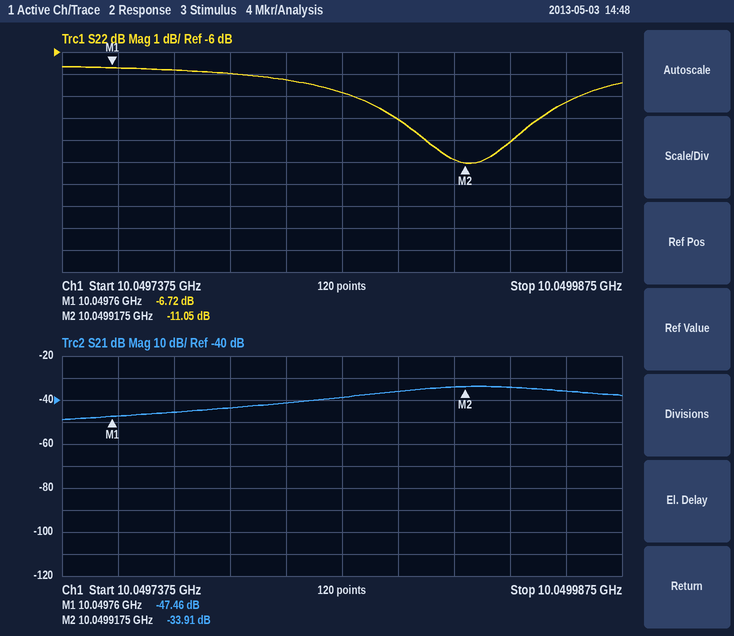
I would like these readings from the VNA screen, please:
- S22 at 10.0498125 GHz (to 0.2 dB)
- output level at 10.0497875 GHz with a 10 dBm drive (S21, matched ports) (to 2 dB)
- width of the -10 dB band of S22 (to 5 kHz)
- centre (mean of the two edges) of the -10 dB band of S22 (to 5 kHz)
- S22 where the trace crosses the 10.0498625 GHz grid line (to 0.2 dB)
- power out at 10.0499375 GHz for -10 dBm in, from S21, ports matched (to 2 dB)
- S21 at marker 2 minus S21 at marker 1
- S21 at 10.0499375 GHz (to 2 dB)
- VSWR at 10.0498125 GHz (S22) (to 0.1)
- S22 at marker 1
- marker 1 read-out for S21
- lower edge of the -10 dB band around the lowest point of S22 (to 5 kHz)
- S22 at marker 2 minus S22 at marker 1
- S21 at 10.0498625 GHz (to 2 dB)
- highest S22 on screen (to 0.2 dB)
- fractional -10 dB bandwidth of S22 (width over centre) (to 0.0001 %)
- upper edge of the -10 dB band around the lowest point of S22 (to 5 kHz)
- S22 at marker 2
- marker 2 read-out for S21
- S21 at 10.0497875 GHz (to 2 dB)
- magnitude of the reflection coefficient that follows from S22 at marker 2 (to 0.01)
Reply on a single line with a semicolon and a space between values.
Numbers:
-7.0 dB; -36 dBm; 40 kHz; 10.049920 GHz; -7.8 dB; -44 dBm; 13.55 dB; -34 dB; 2.6; -6.72 dB; -47.46 dB; 10.049900 GHz; -4.33 dB; -38 dB; -6.6 dB; 0.0004 %; 10.049940 GHz; -11.05 dB; -33.91 dB; -46 dB; 0.28
